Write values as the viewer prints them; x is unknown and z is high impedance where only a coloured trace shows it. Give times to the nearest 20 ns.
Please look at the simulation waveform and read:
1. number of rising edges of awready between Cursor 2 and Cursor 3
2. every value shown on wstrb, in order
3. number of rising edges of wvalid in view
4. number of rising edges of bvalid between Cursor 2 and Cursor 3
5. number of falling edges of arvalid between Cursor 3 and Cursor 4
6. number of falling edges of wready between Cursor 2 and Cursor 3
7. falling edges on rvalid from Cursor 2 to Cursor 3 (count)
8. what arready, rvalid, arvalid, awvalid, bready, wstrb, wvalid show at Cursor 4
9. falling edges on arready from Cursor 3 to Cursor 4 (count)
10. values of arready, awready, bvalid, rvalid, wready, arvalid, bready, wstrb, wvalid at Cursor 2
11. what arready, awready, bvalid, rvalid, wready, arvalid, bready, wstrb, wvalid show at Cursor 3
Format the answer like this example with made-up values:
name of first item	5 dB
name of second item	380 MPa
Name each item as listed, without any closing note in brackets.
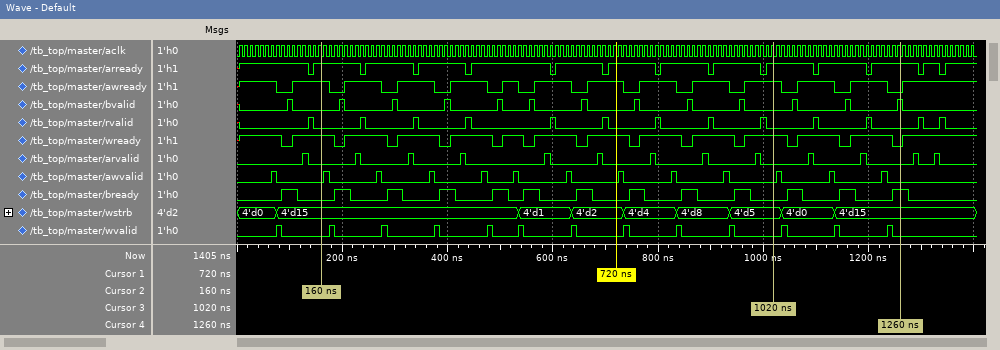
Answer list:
number of rising edges of awready between Cursor 2 and Cursor 3	9
every value shown on wstrb, in order	4'd0, 4'd15, 4'd1, 4'd2, 4'd4, 4'd8, 4'd5, 4'd0, 4'd15
number of rising edges of wvalid in view	13
number of rising edges of bvalid between Cursor 2 and Cursor 3	9
number of falling edges of arvalid between Cursor 3 and Cursor 4	2
number of falling edges of wready between Cursor 2 and Cursor 3	9
falling edges on rvalid from Cursor 2 to Cursor 3	8
what arready, rvalid, arvalid, awvalid, bready, wstrb, wvalid show at Cursor 4	arready=1, rvalid=0, arvalid=0, awvalid=0, bready=1, wstrb=4'd15, wvalid=0
falling edges on arready from Cursor 3 to Cursor 4	2
values of arready, awready, bvalid, rvalid, wready, arvalid, bready, wstrb, wvalid at Cursor 2	arready=1, awready=1, bvalid=0, rvalid=0, wready=1, arvalid=0, bready=0, wstrb=4'd15, wvalid=0
what arready, awready, bvalid, rvalid, wready, arvalid, bready, wstrb, wvalid show at Cursor 3	arready=1, awready=1, bvalid=0, rvalid=0, wready=1, arvalid=0, bready=0, wstrb=4'd5, wvalid=0
